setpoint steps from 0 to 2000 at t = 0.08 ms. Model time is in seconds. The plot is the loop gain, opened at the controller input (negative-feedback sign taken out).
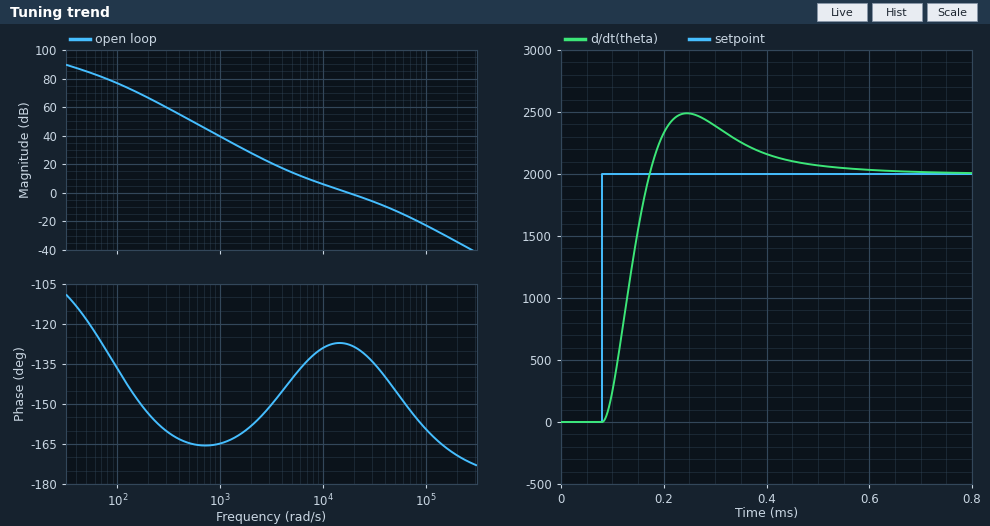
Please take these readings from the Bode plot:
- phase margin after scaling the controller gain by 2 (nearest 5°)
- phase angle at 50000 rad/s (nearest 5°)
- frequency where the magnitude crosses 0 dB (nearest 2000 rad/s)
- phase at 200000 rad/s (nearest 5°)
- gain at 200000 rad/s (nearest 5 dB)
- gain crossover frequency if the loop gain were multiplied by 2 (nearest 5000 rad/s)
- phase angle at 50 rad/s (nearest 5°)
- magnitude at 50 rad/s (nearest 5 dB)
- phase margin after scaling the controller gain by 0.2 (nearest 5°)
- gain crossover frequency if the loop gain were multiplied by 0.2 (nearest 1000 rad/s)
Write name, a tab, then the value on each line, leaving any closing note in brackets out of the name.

phase margin after scaling the controller gain by 2	45°
phase angle at 50000 rad/s	-145°
frequency where the magnitude crosses 0 dB	18000 rad/s
phase at 200000 rad/s	-170°
gain at 200000 rad/s	-35 dB
gain crossover frequency if the loop gain were multiplied by 2	30000 rad/s
phase angle at 50 rad/s	-120°
magnitude at 50 rad/s	85 dB
phase margin after scaling the controller gain by 0.2	40°
gain crossover frequency if the loop gain were multiplied by 0.2	5000 rad/s
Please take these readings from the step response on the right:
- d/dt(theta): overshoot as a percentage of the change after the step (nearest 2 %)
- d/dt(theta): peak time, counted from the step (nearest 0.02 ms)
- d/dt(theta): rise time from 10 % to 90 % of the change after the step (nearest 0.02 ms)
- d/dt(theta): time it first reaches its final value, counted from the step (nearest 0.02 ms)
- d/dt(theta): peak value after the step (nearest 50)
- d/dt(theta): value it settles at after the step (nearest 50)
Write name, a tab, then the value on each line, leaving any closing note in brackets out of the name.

d/dt(theta): overshoot as a percentage of the change after the step	24 %
d/dt(theta): peak time, counted from the step	0.16 ms
d/dt(theta): rise time from 10 % to 90 % of the change after the step	0.06 ms
d/dt(theta): time it first reaches its final value, counted from the step	0.10 ms
d/dt(theta): peak value after the step	2500
d/dt(theta): value it settles at after the step	2000
